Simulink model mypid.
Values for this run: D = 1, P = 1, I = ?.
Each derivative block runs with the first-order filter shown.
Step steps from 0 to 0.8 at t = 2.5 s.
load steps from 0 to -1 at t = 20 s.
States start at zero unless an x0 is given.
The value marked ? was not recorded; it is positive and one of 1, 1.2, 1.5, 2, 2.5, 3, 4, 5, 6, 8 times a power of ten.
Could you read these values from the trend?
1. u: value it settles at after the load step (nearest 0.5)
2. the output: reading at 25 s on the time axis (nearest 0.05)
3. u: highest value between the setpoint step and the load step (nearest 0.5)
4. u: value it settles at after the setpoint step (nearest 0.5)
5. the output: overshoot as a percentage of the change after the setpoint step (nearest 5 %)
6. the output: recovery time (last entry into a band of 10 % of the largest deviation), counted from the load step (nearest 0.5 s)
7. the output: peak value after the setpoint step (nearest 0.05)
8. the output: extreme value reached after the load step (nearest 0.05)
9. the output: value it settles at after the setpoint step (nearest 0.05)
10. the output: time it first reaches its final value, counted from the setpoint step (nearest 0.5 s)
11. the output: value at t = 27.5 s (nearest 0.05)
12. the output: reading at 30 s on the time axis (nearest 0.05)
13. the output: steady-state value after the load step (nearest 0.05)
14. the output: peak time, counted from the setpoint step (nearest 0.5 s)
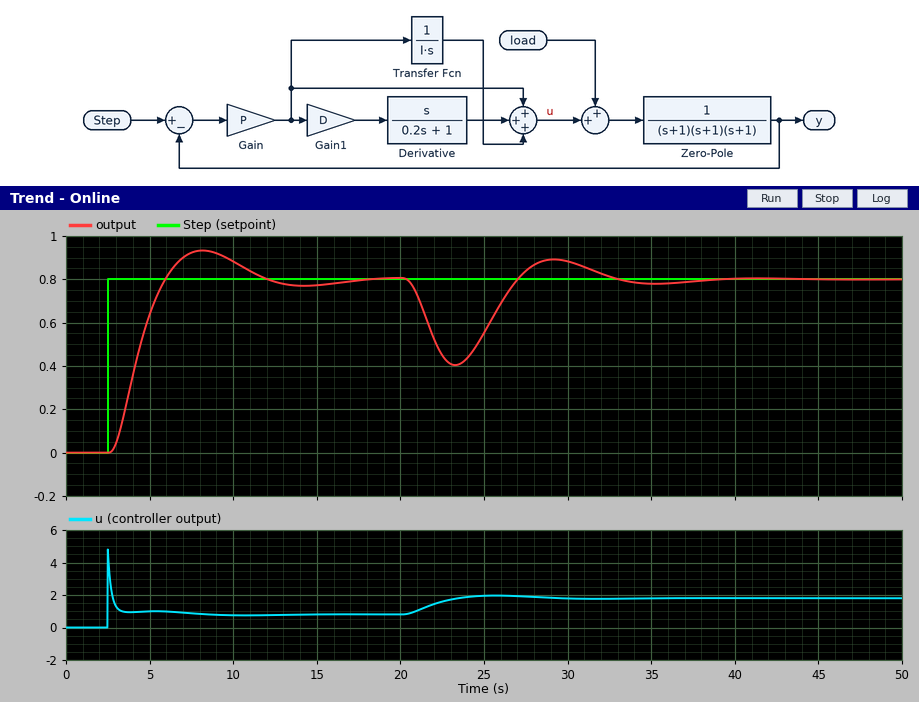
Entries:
2.0
0.55
5.0
1.0
15 %
11.5 s
0.95
0.40
0.80
3.5 s
0.85
0.90
0.80
5.5 s
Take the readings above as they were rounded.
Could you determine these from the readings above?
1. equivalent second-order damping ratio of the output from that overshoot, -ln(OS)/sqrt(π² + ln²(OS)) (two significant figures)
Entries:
0.52
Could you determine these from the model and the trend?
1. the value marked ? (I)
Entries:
1.2
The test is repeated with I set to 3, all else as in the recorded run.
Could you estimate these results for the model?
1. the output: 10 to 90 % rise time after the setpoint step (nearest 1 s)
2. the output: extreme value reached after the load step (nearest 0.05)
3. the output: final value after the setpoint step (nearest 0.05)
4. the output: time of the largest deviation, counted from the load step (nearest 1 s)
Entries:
7 s
0.35
0.80
4 s
